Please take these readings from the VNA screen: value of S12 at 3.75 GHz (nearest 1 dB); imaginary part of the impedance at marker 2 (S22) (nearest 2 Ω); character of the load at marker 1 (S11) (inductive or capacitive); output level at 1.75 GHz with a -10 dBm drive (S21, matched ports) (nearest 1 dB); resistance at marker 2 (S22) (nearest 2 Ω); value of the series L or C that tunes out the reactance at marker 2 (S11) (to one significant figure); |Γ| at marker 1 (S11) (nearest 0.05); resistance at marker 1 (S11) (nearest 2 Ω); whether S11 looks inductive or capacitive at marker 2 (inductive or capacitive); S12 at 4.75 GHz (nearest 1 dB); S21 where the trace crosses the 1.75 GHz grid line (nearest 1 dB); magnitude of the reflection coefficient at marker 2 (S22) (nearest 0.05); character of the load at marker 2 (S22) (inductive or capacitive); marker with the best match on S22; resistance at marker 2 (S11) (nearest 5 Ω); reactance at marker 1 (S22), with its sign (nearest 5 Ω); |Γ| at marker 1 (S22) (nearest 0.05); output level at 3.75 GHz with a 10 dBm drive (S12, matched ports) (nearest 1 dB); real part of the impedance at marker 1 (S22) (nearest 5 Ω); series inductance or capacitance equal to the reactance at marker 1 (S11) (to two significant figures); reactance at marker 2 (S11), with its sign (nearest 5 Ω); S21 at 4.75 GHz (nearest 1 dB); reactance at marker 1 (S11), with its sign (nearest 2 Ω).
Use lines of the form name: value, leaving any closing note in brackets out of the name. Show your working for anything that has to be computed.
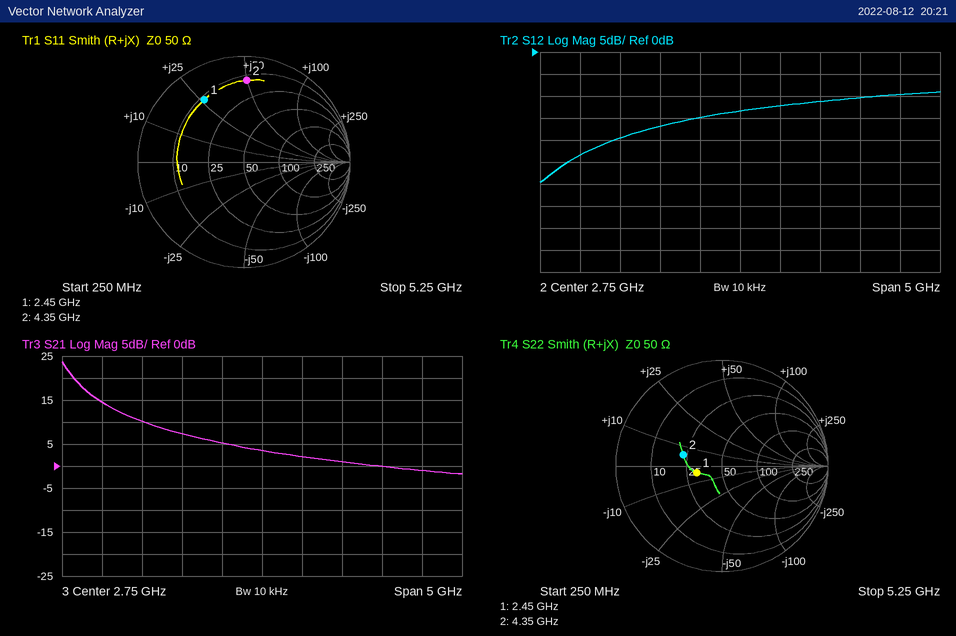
value of S12 at 3.75 GHz: -11 dB
imaginary part of the impedance at marker 2 (S22): +6 Ω
character of the load at marker 1 (S11): inductive
output level at 1.75 GHz with a -10 dBm drive (S21, matched ports): -10 dBm + (7 dB) = -3 dBm
resistance at marker 2 (S22): 22 Ω
value of the series L or C that tunes out the reactance at marker 2 (S11): C = 1/(2π × 4.35 GHz × 50 Ω) ≈ 732 fF, so 700 fF to one significant figure
|Γ| at marker 1 (S11): 0.70
resistance at marker 1 (S11): 12 Ω
whether S11 looks inductive or capacitive at marker 2: inductive
S12 at 4.75 GHz: -10 dB
S21 where the trace crosses the 1.75 GHz grid line: 7 dB
magnitude of the reflection coefficient at marker 2 (S22): 0.40
character of the load at marker 2 (S22): inductive
marker with the best match on S22: marker 1
resistance at marker 2 (S11): 15 Ω
reactance at marker 1 (S22), with its sign: -5 Ω
|Γ| at marker 1 (S22): 0.25
output level at 3.75 GHz with a 10 dBm drive (S12, matched ports): 10 dBm + (-11 dB) = -1 dBm
real part of the impedance at marker 1 (S22): 30 Ω
series inductance or capacitance equal to the reactance at marker 1 (S11): L = 26 Ω/(2π × 2.45 GHz) ≈ 1.7 nH
reactance at marker 2 (S11), with its sign: +50 Ω
S21 at 4.75 GHz: -1 dB
reactance at marker 1 (S11), with its sign: +26 Ω
